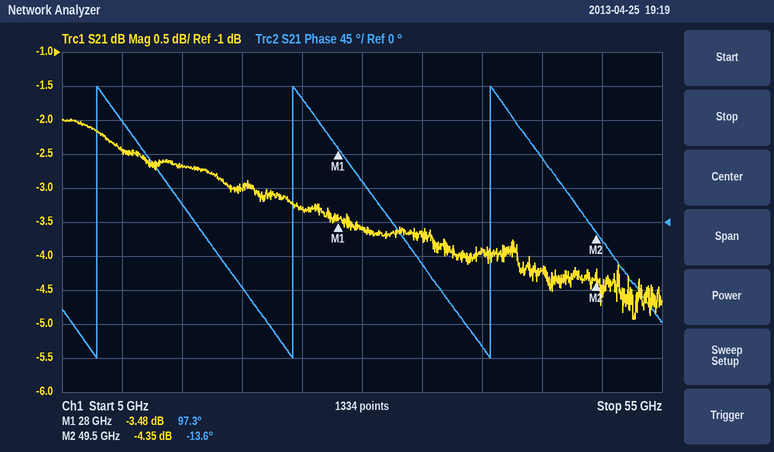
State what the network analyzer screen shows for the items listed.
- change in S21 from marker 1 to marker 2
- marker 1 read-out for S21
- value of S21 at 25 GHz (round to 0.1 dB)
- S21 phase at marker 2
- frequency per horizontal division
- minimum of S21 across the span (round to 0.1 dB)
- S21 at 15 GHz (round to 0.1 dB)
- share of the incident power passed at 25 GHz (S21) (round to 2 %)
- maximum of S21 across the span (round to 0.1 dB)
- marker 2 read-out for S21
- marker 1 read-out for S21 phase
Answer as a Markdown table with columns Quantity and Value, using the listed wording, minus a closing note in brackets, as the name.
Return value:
| Quantity | Value |
|---|---|
| change in S21 from marker 1 to marker 2 | -0.87 dB |
| marker 1 read-out for S21 | -3.48 dB |
| value of S21 at 25 GHz | -3.3 dB |
| S21 phase at marker 2 | -13.6° |
| frequency per horizontal division | 5 GHz |
| minimum of S21 across the span | -4.9 dB |
| S21 at 15 GHz | -2.7 dB |
| share of the incident power passed at 25 GHz (S21) | 46 % |
| maximum of S21 across the span | -2.0 dB |
| marker 2 read-out for S21 | -4.35 dB |
| marker 1 read-out for S21 phase | 97.3° |
